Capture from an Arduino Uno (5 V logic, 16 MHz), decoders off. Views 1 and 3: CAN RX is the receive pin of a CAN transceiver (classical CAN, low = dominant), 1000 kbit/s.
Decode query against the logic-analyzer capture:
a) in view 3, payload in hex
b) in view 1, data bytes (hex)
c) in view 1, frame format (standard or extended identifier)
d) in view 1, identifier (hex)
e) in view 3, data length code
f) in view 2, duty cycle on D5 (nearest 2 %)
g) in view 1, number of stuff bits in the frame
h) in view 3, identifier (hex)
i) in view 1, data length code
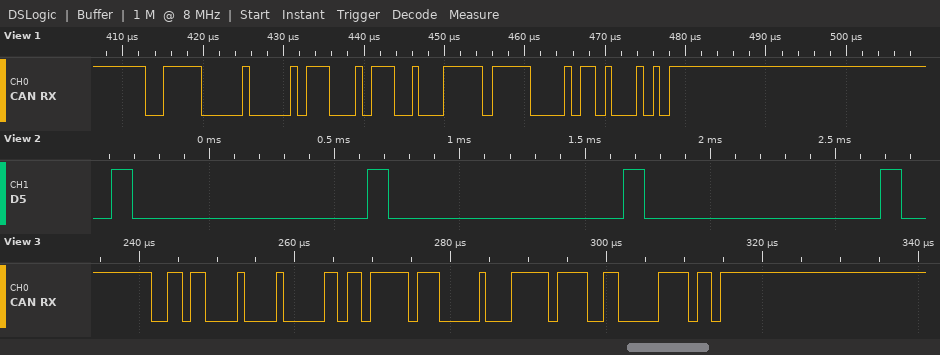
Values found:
16 FF 00 FF
8B 91 FF
standard
0x3E0
4
8 %
5
0x361
3
